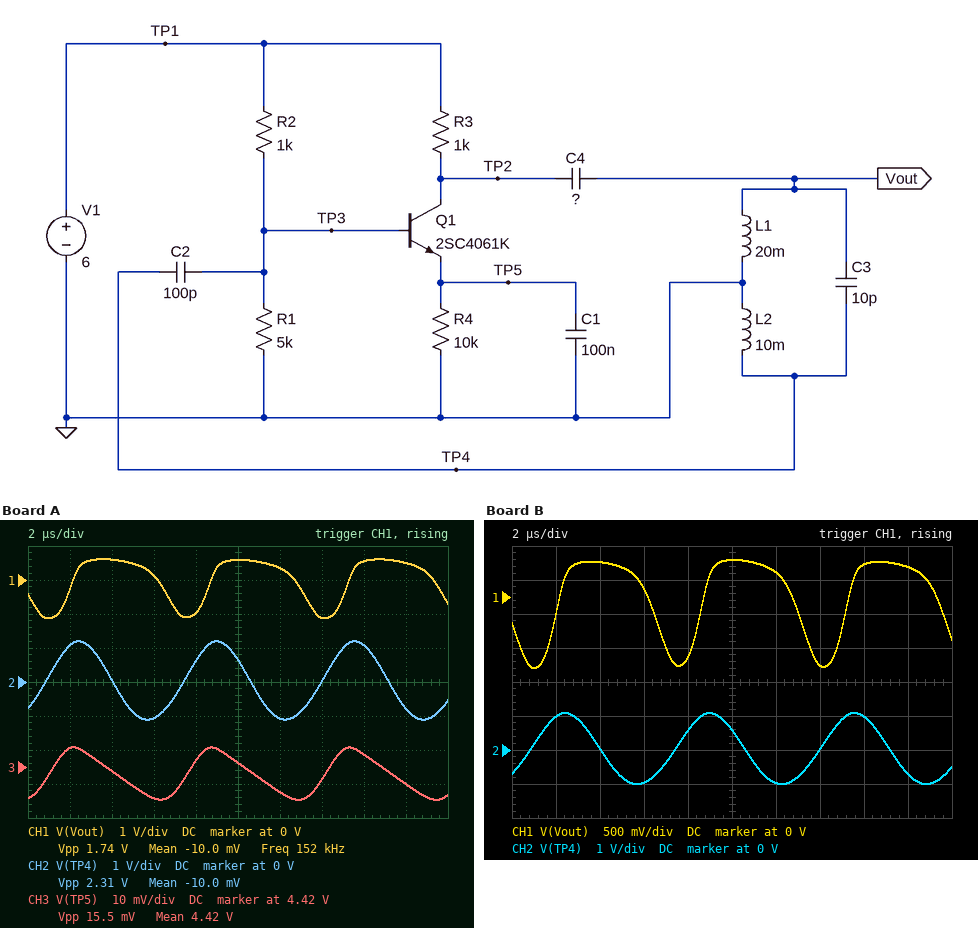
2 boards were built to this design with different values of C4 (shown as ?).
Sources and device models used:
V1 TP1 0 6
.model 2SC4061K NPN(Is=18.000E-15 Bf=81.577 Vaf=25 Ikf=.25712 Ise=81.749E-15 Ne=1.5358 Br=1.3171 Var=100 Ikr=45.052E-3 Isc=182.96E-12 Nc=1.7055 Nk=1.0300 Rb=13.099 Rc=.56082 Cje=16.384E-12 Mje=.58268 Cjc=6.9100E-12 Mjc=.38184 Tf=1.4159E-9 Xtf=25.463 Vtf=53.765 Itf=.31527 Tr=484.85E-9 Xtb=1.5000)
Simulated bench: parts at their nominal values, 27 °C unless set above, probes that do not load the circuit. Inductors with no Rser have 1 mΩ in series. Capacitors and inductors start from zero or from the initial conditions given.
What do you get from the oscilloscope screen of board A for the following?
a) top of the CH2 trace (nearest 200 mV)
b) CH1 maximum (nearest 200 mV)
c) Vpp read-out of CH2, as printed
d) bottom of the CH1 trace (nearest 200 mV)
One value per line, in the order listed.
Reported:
1.2 V
600 mV
2.31 V
-1.2 V
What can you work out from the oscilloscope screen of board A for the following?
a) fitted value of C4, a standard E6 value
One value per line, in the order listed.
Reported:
220 pF
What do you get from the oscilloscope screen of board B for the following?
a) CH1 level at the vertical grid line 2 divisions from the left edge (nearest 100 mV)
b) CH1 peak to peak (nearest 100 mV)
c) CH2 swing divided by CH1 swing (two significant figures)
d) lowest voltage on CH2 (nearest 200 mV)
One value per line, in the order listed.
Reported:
500 mV
1.6 V
1.3
-1.0 V
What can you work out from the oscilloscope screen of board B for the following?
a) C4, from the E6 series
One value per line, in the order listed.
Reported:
330 pF
